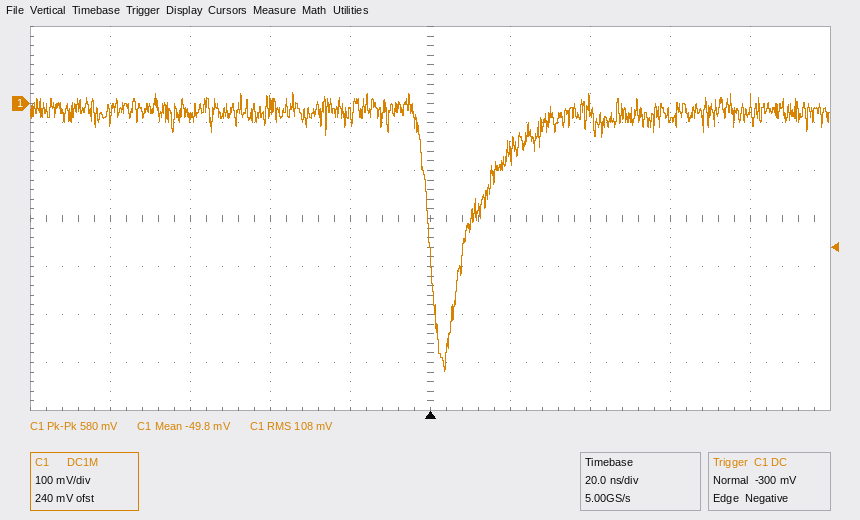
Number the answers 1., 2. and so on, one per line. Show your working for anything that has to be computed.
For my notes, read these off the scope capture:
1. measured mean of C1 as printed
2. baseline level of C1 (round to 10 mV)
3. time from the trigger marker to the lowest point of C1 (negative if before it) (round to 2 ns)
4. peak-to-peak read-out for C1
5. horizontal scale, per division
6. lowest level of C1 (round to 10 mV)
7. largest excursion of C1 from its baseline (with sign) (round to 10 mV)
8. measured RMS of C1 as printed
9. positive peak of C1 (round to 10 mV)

1. -49.8 mV
2. -20 mV
3. +4 ns
4. 580 mV
5. 20 ns
6. -560 mV
7. -560 mV − (-20 mV) = -540 mV
8. 108 mV
9. 20 mV
